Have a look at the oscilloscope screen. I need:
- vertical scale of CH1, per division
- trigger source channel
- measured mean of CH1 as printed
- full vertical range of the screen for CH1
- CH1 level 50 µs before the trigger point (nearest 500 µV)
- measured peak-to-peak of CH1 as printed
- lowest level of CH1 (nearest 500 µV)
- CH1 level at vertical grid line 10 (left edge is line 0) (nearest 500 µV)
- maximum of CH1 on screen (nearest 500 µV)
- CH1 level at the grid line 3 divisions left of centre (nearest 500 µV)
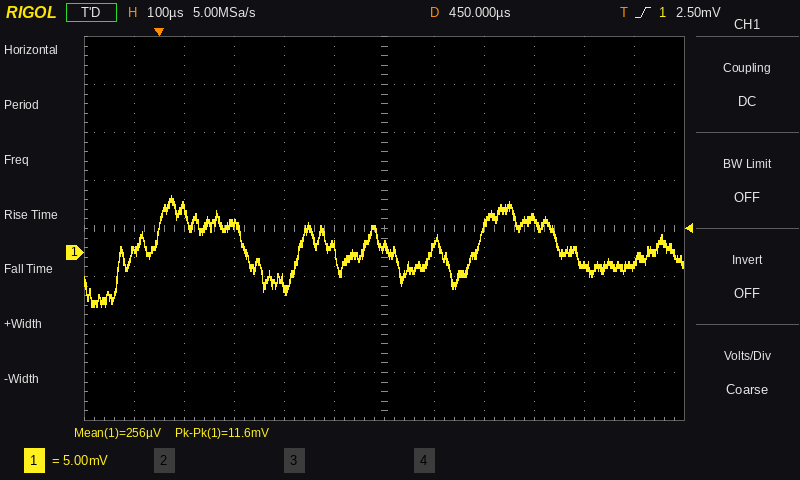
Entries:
5 mV
CH1
256 µV
40 mV
0.0 mV
11.6 mV
-5.5 mV
-1.5 mV
6.0 mV
3.0 mV
